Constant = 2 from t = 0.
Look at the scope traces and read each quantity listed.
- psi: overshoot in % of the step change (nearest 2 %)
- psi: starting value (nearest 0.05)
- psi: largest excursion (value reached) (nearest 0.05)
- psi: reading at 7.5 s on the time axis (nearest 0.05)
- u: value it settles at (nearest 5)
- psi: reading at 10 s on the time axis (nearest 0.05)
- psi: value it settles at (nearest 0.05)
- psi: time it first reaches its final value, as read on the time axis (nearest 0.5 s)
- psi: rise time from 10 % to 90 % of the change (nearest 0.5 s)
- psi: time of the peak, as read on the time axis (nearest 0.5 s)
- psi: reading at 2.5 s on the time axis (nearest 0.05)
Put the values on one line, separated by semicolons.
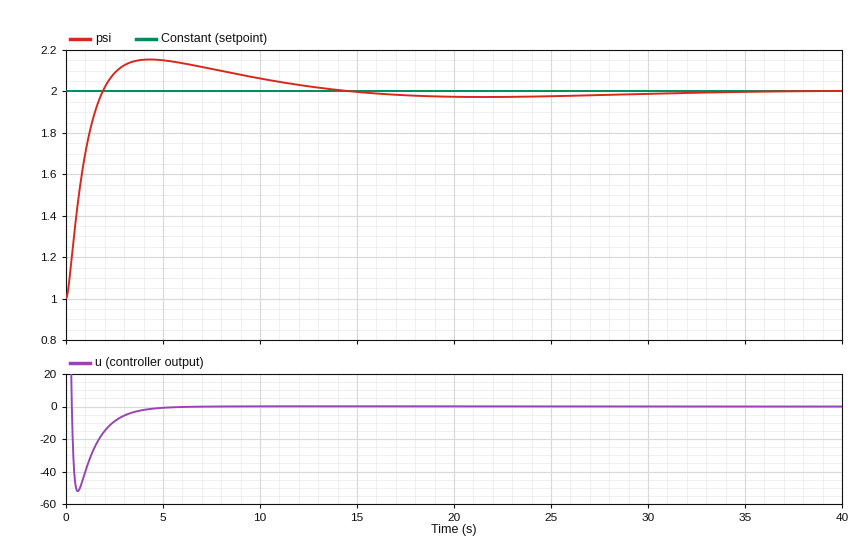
16 %; 1.00; 2.15; 2.10; 0; 2.05; 2.00; 2.0 s; 1.5 s; 4.5 s; 2.10
